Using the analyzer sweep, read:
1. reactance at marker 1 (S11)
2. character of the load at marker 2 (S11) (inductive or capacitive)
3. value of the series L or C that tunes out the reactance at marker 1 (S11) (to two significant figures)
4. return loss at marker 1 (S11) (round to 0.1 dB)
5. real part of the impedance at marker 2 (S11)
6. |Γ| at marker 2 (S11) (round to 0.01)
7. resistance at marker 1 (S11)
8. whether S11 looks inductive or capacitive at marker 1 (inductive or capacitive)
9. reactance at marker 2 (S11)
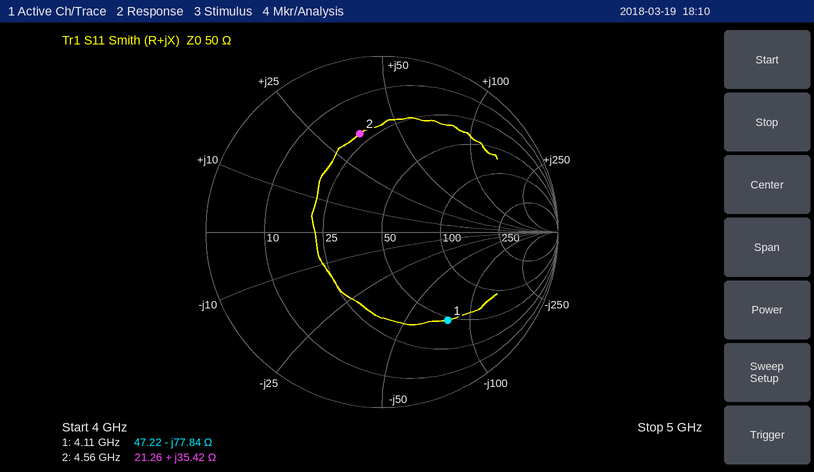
-77.84 Ω
inductive
3.0 nH
4.1 dB
21.26 Ω
0.57
47.22 Ω
capacitive
+35.42 Ω
